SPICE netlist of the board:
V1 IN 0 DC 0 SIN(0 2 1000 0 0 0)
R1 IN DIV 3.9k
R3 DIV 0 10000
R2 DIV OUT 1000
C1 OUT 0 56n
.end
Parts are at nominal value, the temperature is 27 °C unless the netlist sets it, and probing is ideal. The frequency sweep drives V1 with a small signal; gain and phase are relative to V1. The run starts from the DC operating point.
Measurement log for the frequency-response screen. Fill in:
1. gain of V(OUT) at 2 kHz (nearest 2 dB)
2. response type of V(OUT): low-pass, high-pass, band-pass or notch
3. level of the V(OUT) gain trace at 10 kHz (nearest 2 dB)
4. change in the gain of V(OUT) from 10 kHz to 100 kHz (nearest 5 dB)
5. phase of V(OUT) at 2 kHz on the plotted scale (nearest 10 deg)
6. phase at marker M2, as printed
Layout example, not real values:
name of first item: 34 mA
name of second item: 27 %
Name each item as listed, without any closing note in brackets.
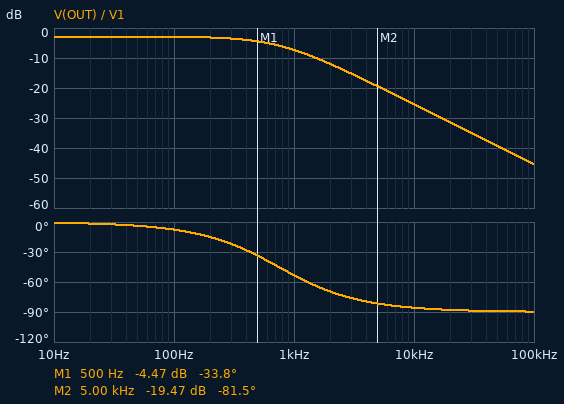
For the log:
gain of V(OUT) at 2 kHz: -12 dB
response type of V(OUT): low-pass, high-pass, band-pass or notch: low-pass
level of the V(OUT) gain trace at 10 kHz: -26 dB
change in the gain of V(OUT) from 10 kHz to 100 kHz: -20 dB
phase of V(OUT) at 2 kHz on the plotted scale: -70 deg
phase at marker M2, as printed: -81.5 deg
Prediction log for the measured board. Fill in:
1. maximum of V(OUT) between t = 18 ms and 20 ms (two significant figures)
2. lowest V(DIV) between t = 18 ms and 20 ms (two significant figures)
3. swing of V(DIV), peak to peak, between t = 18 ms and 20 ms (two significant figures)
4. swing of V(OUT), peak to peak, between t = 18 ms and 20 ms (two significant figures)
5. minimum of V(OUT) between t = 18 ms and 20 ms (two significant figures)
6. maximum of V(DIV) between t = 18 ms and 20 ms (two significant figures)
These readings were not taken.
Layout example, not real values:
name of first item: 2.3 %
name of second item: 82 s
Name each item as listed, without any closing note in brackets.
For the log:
maximum of V(OUT) between t = 18 ms and 20 ms: 860 mV
lowest V(DIV) between t = 18 ms and 20 ms: -910 mV
swing of V(DIV), peak to peak, between t = 18 ms and 20 ms: 1.8 V
swing of V(OUT), peak to peak, between t = 18 ms and 20 ms: 1.7 V
minimum of V(OUT) between t = 18 ms and 20 ms: -860 mV
maximum of V(DIV) between t = 18 ms and 20 ms: 910 mV
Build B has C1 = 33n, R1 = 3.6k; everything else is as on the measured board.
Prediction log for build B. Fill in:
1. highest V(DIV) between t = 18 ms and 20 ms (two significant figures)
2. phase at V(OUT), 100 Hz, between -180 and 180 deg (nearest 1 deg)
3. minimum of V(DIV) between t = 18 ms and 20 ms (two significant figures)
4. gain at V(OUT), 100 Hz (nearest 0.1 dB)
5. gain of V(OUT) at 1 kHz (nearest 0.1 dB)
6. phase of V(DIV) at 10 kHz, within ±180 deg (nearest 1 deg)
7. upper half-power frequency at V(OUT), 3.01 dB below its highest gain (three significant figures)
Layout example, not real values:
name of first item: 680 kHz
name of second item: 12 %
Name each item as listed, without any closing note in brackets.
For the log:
highest V(DIV) between t = 18 ms and 20 ms: 1.2 V
phase at V(OUT), 100 Hz, between -180 and 180 deg: -4 deg
minimum of V(DIV) between t = 18 ms and 20 ms: -1.2 V
gain at V(OUT), 100 Hz: -2.7 dB
gain of V(OUT) at 1 kHz: -4.6 dB
phase of V(DIV) at 10 kHz, within ±180 deg: -18 deg
upper half-power frequency at V(OUT), 3.01 dB below its highest gain: 1.32 kHz
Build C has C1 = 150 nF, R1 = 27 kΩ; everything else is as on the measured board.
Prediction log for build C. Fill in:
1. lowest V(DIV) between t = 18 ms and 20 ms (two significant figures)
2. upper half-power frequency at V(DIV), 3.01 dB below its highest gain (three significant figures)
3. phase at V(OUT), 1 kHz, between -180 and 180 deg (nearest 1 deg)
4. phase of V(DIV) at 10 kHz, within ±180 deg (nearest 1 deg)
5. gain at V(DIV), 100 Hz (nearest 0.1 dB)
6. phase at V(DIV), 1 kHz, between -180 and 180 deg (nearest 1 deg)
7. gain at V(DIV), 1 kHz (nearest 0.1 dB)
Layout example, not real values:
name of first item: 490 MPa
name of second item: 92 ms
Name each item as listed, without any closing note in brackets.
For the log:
lowest V(DIV) between t = 18 ms and 20 ms: -94 mV
upper half-power frequency at V(DIV), 3.01 dB below its highest gain: 130 Hz
phase at V(OUT), 1 kHz, between -180 and 180 deg: -83 deg
phase of V(DIV) at 10 kHz, within ±180 deg: -5 deg
gain at V(DIV), 100 Hz: -13.4 dB
phase at V(DIV), 1 kHz, between -180 and 180 deg: -39 deg
gain at V(DIV), 1 kHz: -26.5 dB
